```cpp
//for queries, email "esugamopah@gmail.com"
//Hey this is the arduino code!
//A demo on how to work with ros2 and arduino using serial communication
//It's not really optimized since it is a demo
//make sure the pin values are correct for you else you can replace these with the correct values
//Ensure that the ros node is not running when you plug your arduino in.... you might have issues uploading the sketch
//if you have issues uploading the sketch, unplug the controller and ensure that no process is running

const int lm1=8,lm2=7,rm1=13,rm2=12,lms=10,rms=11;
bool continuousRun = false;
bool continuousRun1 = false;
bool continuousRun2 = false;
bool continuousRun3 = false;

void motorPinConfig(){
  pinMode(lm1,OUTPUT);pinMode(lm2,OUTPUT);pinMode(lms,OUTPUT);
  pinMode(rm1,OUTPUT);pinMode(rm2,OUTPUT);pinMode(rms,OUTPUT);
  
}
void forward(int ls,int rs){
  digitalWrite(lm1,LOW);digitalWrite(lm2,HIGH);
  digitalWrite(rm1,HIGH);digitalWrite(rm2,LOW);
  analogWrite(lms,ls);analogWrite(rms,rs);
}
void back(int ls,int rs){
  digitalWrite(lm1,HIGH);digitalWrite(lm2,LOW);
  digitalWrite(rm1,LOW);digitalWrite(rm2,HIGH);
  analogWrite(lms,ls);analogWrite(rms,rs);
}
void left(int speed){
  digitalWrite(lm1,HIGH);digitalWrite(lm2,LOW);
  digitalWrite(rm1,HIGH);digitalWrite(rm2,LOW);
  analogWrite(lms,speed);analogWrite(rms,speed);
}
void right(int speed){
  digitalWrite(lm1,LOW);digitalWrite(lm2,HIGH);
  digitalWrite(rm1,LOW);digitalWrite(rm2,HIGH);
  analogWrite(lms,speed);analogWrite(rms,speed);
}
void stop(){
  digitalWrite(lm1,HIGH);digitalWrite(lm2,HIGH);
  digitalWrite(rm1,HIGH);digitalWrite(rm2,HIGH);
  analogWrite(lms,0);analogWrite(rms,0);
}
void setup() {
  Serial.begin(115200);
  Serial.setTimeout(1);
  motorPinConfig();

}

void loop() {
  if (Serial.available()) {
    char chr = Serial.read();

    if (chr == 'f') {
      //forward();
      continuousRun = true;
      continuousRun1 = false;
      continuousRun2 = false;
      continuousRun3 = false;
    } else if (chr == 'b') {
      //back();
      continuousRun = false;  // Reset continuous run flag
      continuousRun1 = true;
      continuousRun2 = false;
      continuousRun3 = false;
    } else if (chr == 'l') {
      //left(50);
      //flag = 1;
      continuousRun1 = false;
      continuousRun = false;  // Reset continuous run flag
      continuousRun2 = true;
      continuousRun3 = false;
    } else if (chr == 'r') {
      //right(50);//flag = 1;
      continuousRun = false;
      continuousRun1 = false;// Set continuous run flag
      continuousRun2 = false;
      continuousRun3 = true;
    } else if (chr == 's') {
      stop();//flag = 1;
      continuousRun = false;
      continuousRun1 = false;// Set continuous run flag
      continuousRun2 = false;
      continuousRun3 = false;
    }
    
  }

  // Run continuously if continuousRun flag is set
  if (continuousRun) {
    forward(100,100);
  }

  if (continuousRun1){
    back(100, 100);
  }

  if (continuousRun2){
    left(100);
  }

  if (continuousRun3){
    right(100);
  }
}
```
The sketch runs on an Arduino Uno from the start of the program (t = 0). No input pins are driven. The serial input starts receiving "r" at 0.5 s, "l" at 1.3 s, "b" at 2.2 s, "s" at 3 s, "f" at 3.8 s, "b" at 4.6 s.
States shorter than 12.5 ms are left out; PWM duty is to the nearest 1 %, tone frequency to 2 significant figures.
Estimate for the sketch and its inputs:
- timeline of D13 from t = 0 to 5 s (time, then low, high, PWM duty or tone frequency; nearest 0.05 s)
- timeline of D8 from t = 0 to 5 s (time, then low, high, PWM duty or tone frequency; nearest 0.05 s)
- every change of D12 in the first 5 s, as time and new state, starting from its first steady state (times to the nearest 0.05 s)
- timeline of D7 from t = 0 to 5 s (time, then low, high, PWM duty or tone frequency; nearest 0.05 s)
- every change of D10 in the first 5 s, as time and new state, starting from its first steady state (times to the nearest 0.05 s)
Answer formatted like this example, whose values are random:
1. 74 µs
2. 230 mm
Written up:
1. 0 s low; 1.3 s high; 2.2 s low; 3 s high; 4.6 s low
2. 0 s low; 1.3 s high; 3.8 s low; 4.6 s high
3. 0 s low; 0.5 s high; 1.3 s low; 2.2 s high; 3.8 s low; 4.6 s high
4. 0 s low; 0.5 s high; 1.3 s low; 3 s high; 4.6 s low
5. 0 s low; 0.5 s PWM 39 %; 3 s low; 3.8 s PWM 39 %
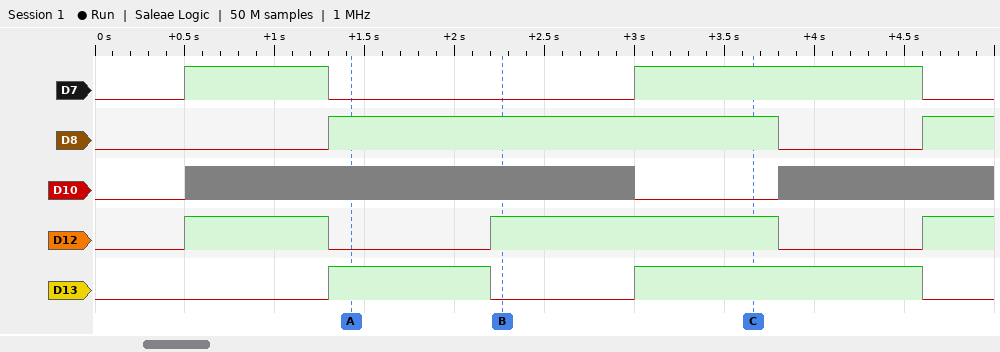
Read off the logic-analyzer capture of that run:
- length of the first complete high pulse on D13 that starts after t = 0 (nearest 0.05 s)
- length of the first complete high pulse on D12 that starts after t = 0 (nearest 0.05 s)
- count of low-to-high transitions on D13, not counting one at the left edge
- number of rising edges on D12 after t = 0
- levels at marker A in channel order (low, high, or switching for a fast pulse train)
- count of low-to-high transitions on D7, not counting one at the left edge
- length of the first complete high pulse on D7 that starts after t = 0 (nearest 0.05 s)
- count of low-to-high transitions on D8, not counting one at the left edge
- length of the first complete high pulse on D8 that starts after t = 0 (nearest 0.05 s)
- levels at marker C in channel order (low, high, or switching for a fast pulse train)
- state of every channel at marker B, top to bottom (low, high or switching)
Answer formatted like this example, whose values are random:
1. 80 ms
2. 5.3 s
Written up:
1. 0.90 s
2. 0.80 s
3. 2
4. 3
5. D7 low, D8 high, D10 switching, D12 low, D13 high
6. 2
7. 0.80 s
8. 2
9. 2.50 s
10. D7 high, D8 high, D10 low, D12 high, D13 high
11. D7 low, D8 high, D10 switching, D12 high, D13 low
